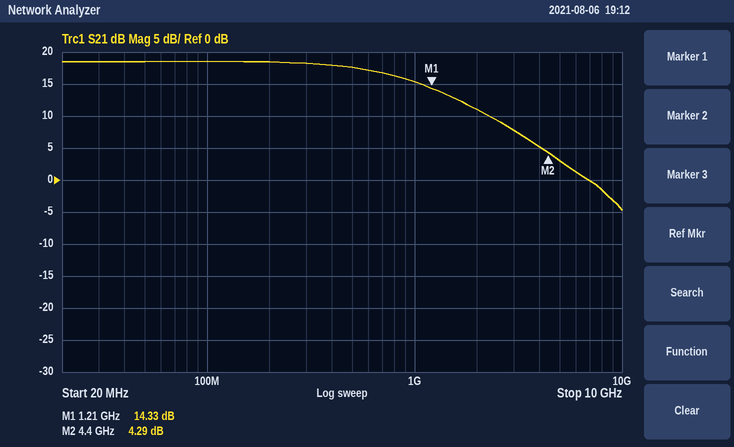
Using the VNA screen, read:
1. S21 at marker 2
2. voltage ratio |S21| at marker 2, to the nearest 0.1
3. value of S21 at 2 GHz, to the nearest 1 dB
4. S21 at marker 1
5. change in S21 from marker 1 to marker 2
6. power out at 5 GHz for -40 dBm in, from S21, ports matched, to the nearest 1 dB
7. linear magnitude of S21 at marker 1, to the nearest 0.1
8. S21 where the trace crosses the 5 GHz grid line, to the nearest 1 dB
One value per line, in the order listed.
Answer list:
4.29 dB
1.6
11 dB
14.33 dB
-10.04 dB
-37 dBm
5.2
3 dB
